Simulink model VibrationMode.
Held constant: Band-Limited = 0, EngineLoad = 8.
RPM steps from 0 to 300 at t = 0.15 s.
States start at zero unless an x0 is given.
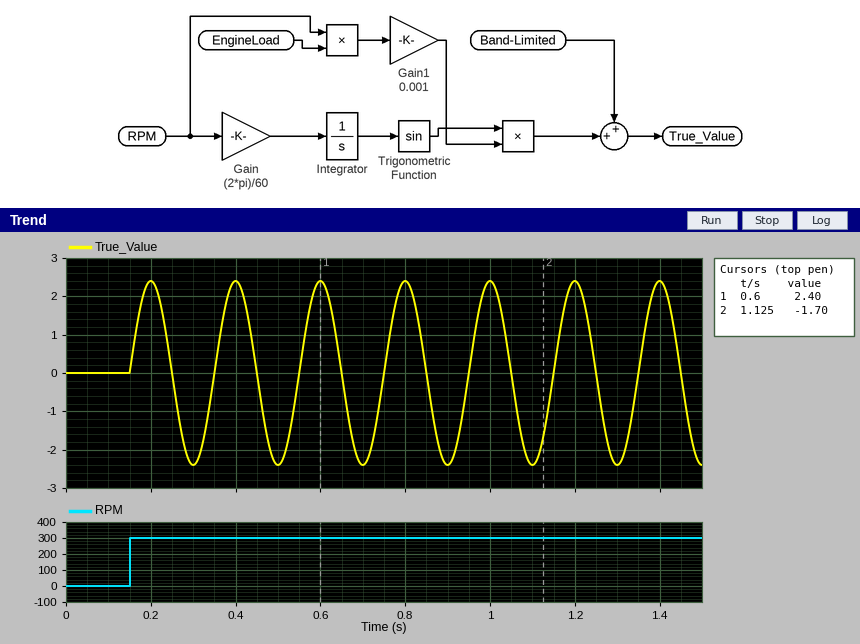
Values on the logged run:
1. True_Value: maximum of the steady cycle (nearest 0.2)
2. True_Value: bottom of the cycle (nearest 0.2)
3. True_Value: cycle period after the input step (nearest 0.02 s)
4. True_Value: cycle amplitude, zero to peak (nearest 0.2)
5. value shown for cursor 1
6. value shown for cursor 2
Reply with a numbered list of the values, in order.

1. 2.4
2. -2.4
3. 0.20 s
4. 2.4
5. 2.40
6. -1.70
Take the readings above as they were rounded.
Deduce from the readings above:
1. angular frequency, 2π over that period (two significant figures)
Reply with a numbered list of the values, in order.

1. 31 rad/s
